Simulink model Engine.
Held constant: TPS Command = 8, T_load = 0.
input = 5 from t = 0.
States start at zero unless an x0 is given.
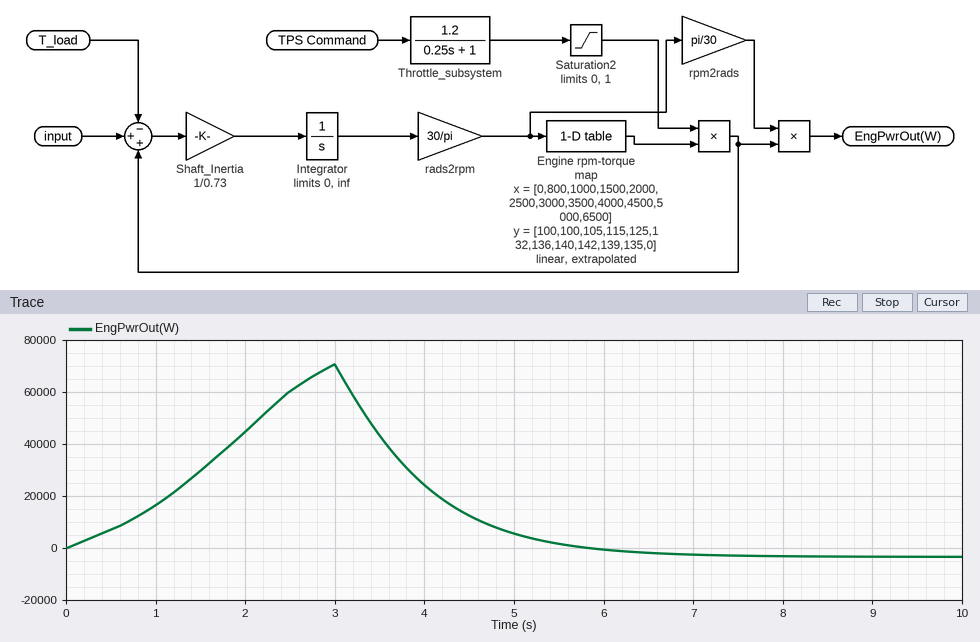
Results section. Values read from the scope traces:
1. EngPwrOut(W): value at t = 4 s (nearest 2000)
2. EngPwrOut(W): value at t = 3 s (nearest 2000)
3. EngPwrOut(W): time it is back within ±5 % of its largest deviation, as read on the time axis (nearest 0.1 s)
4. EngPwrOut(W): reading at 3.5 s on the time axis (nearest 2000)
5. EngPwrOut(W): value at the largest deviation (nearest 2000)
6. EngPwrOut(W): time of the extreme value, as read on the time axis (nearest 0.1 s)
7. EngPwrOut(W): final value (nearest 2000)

24000
70000
5.8 s
44000
70000
3.0 s
-4000
